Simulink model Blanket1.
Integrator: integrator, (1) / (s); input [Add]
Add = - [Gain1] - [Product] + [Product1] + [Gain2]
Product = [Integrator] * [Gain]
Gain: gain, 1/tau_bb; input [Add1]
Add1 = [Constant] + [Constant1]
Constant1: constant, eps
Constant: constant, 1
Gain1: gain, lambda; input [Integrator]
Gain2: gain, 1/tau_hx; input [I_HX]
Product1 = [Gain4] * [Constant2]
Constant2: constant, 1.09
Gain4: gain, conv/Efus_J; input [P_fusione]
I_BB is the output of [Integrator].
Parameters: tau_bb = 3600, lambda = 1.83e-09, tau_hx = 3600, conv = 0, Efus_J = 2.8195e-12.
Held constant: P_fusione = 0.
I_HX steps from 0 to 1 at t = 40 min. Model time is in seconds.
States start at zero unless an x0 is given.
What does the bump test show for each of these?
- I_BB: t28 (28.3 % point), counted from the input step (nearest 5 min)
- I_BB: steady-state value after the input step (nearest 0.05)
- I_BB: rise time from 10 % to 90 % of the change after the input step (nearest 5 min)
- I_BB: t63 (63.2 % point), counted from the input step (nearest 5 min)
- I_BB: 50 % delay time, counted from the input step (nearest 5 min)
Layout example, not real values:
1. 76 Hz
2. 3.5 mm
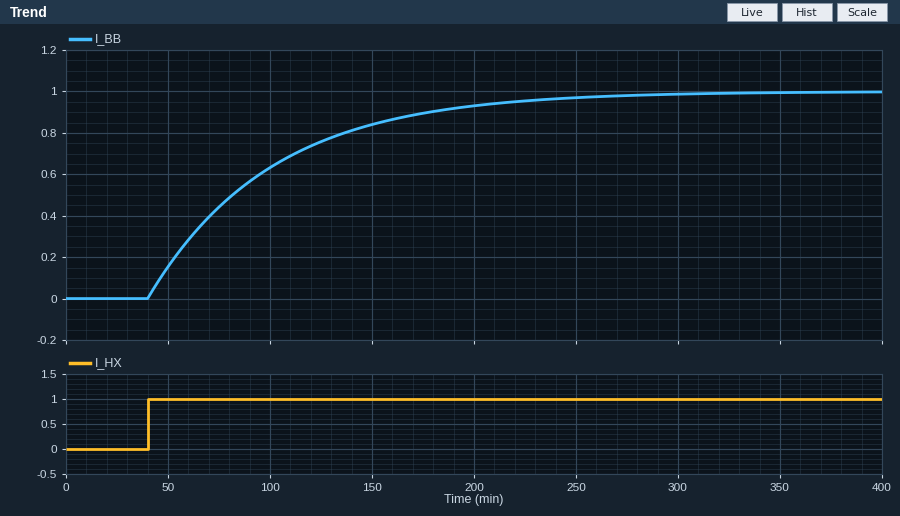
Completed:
1. 20 min
2. 1.00
3. 130 min
4. 60 min
5. 40 min
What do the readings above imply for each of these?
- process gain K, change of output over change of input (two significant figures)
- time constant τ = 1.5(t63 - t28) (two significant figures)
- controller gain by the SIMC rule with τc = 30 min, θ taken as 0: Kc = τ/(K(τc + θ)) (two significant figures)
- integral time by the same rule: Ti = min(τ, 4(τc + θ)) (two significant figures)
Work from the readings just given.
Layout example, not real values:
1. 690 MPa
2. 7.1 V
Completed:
1. 1.0
2. 60 min
3. 2.0
4. 60 min
